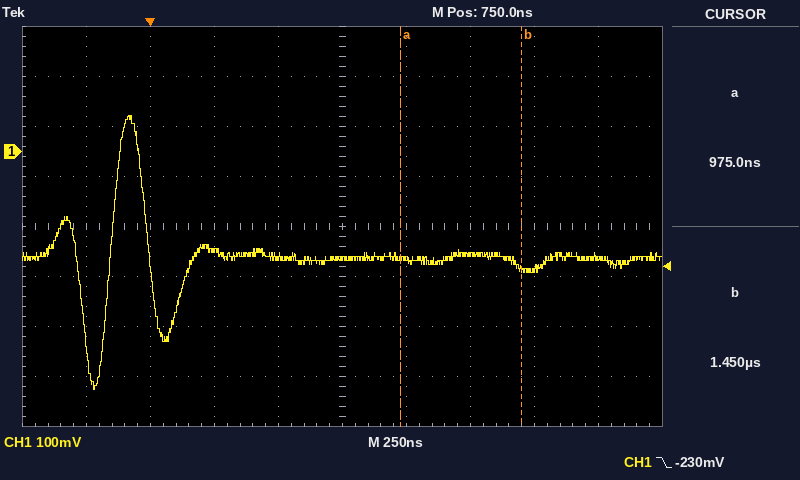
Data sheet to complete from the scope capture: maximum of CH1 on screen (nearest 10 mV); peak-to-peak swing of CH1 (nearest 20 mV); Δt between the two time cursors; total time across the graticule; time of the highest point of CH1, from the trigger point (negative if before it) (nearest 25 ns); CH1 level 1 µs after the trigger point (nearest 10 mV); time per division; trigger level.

70 mV
540 mV
475 ns
2.5 µs
-75 ns
-220 mV
250 ns
-230 mV
